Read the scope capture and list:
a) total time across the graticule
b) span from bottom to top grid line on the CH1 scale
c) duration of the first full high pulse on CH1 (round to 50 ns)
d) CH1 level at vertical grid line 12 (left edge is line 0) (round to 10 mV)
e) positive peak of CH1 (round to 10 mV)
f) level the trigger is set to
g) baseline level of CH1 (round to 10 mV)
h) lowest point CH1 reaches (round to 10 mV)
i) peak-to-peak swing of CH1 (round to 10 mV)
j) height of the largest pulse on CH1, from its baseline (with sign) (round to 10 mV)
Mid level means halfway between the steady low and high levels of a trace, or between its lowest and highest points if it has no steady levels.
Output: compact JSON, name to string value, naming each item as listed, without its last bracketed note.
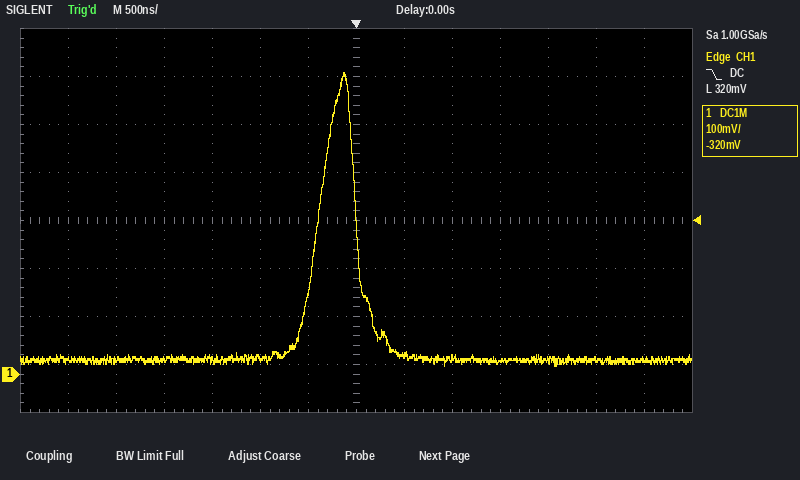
{"total time across the graticule": "7 µs", "span from bottom to top grid line on the CH1 scale": "800 mV", "duration of the first full high pulse on CH1": "400 ns", "CH1 level at vertical grid line 12 (left edge is line 0)": "30 mV", "positive peak of CH1": "630 mV", "level the trigger is set to": "320 mV", "baseline level of CH1": "30 mV", "lowest point CH1 reaches": "20 mV", "peak-to-peak swing of CH1": "610 mV", "height of the largest pulse on CH1, from its baseline (with sign)": "+600 mV"}
